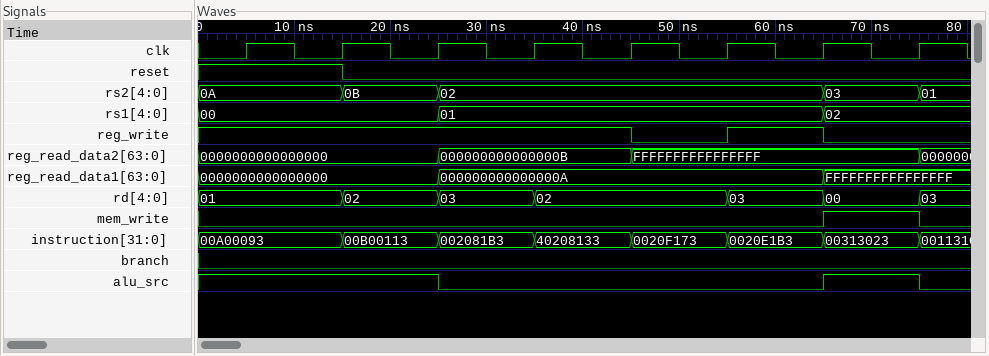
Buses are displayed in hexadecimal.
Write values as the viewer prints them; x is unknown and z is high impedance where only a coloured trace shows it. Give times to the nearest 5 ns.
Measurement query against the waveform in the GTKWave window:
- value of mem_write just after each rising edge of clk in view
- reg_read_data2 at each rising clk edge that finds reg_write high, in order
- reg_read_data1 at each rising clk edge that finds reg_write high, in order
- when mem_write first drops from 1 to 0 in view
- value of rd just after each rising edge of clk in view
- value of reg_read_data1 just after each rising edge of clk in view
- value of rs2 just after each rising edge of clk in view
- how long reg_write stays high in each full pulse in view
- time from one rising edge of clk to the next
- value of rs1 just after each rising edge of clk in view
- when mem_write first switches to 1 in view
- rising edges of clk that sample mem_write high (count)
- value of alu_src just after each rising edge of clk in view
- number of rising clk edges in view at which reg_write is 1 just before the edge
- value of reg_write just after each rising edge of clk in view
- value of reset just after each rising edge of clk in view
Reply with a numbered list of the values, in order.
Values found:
1. 0 0 0 0 0 0 1 0
2. 0000000000000000, 0000000000000000, 0000000000000000, 000000000000000B, 000000000000000B, FFFFFFFFFFFFFFFF
3. 0000000000000000, 0000000000000000, 0000000000000000, 000000000000000A, 000000000000000A, 000000000000000A
4. 75 ns
5. 01, 02, 03, 02, 02, 03, 00, 03
6. 0000000000000000, 0000000000000000, 000000000000000A, 000000000000000A, 000000000000000A, 000000000000000A, FFFFFFFFFFFFFFFF, FFFFFFFFFFFFFFFF
7. 0A, 0B, 02, 02, 02, 02, 03, 01
8. 10 ns
9. 10 ns
10. 00, 00, 01, 01, 01, 01, 02, 02
11. 65 ns
12. 1
13. 1 1 0 0 0 0 1 0
14. 6
15. 1 1 1 1 0 1 0 0
16. 1 0 0 0 0 0 0 0
